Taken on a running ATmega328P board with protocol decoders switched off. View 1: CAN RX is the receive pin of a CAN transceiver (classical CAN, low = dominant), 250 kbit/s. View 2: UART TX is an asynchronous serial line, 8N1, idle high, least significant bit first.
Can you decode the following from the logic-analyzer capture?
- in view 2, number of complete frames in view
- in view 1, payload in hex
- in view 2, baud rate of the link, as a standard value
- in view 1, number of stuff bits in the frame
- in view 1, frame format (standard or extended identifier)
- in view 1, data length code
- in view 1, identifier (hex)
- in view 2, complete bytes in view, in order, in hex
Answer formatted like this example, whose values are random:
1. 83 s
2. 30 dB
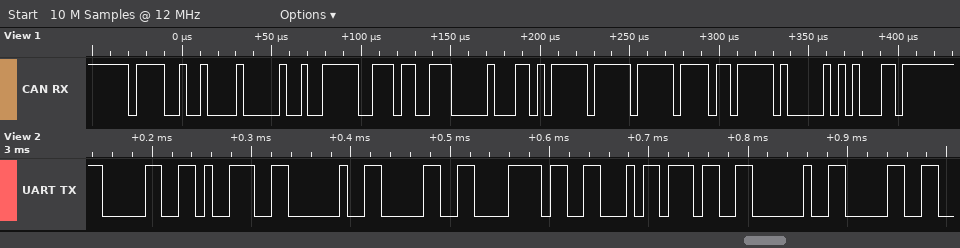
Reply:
1. 9
2. 09 F7 67 00 D7 FF FF 6F
3. 115200 baud
4. 8
5. standard
6. 8
7. 0x792
8. 30 39 20 30 78 46 37 20 30
